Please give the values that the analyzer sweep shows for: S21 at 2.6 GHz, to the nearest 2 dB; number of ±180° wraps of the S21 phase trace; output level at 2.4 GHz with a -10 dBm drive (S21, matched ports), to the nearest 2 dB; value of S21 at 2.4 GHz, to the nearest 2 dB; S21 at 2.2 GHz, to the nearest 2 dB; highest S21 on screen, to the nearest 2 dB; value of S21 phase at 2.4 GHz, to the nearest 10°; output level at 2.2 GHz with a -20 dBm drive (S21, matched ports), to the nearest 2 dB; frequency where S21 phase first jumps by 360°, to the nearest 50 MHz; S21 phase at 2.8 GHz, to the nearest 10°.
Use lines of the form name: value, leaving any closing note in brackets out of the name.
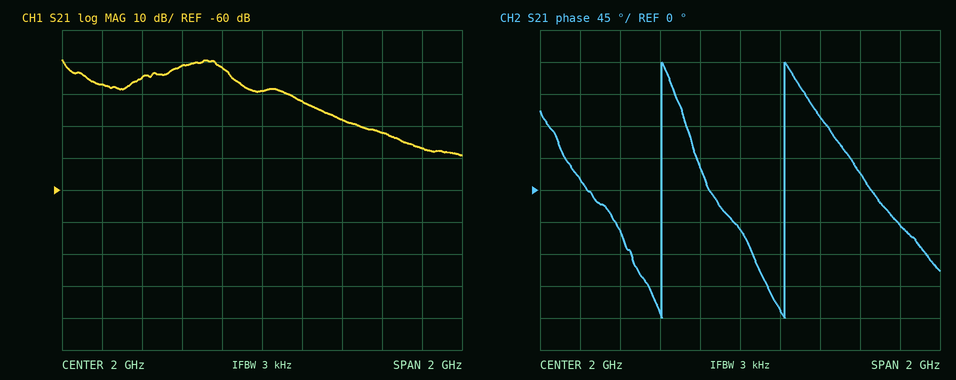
S21 at 2.6 GHz, to the nearest 2 dB: -42 dB
number of ±180° wraps of the S21 phase trace: 2
output level at 2.4 GHz with a -10 dBm drive (S21, matched ports), to the nearest 2 dB: -48 dBm
value of S21 at 2.4 GHz, to the nearest 2 dB: -38 dB
S21 at 2.2 GHz, to the nearest 2 dB: -32 dB
highest S21 on screen, to the nearest 2 dB: -20 dB
value of S21 phase at 2.4 GHz, to the nearest 10°: 100°
output level at 2.2 GHz with a -20 dBm drive (S21, matched ports), to the nearest 2 dB: -52 dBm
frequency where S21 phase first jumps by 360°, to the nearest 50 MHz: 1.60 GHz
S21 phase at 2.8 GHz, to the nearest 10°: -50°
